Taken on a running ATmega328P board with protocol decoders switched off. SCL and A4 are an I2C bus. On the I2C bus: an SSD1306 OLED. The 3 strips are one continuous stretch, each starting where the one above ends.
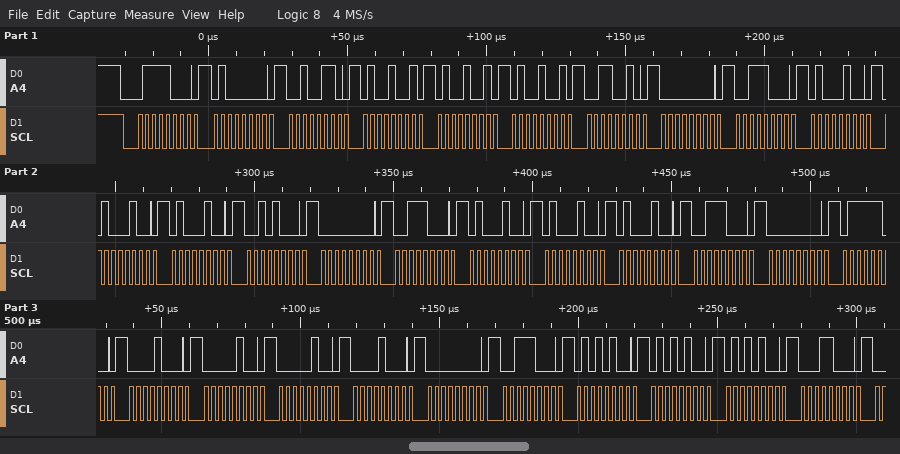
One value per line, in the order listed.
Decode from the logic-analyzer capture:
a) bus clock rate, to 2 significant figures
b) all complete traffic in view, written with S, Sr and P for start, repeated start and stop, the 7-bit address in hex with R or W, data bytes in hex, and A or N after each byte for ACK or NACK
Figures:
400 kHz
S 3CW A 40 A 26 A 49 A 49 A 49 A 32 A 00 A 38 A 44 A 44 A 44 A 28 A 00 A 38 A 44 A 44 A 44 A 38 A 00 A 7C A 08 A 04 A 04 A 08 A 00 A 38 A 54 A 54 A 54 A 18 A
